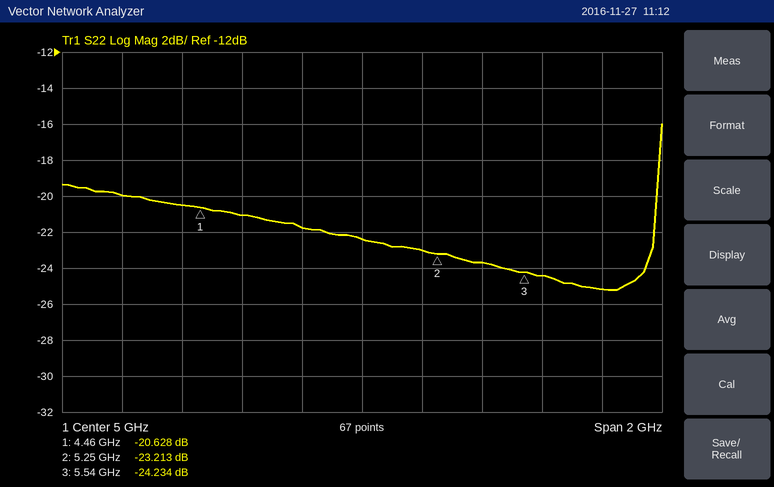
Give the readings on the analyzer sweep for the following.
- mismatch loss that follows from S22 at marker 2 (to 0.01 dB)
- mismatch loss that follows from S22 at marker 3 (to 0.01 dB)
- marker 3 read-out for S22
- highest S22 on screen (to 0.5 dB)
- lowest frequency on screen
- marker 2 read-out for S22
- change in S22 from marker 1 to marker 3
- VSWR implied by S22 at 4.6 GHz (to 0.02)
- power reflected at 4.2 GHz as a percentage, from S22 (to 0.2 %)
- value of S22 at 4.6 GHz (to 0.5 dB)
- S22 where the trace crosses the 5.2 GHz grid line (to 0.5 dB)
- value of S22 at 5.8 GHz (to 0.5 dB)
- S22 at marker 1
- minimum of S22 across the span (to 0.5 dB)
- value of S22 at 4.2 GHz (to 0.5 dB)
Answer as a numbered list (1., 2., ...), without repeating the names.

1. 0.02 dB
2. 0.02 dB
3. -24.234 dB
4. -16.0 dB
5. 4 GHz
6. -23.213 dB
7. -3.606 dB
8. 1.20
9. 1.0 %
10. -21.0 dB
11. -23.0 dB
12. -25.0 dB
13. -20.628 dB
14. -25.0 dB
15. -20.0 dB
